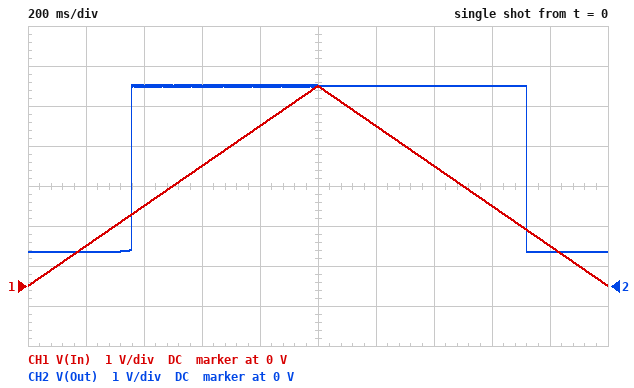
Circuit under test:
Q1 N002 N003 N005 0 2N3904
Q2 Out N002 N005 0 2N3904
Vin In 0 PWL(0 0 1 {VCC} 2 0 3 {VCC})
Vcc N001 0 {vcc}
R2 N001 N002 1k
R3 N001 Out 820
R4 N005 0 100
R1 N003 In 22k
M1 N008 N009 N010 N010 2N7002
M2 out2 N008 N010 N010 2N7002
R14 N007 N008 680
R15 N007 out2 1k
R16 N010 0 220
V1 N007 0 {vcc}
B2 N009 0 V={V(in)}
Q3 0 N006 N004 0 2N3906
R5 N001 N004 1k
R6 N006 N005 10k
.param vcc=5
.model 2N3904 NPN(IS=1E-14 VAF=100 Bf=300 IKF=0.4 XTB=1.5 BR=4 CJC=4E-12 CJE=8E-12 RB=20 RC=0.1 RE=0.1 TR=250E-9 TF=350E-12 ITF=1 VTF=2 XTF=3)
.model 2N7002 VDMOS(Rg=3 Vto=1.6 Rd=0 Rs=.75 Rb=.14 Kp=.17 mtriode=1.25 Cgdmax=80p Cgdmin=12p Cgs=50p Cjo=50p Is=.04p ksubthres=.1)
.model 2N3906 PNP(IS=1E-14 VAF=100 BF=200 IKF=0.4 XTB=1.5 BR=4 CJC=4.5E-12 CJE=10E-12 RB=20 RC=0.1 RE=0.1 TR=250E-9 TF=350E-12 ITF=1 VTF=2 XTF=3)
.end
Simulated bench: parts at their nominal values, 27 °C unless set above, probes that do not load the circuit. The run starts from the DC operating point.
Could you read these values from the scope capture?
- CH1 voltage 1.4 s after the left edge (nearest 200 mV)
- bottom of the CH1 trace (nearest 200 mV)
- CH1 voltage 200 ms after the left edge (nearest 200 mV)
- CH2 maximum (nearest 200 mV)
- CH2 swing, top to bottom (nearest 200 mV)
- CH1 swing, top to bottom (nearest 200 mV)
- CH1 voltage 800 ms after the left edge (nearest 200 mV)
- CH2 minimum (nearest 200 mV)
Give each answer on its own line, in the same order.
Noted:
3.0 V
0 V
1.0 V
5.0 V
4.2 V
5.0 V
4.0 V
800 mV
